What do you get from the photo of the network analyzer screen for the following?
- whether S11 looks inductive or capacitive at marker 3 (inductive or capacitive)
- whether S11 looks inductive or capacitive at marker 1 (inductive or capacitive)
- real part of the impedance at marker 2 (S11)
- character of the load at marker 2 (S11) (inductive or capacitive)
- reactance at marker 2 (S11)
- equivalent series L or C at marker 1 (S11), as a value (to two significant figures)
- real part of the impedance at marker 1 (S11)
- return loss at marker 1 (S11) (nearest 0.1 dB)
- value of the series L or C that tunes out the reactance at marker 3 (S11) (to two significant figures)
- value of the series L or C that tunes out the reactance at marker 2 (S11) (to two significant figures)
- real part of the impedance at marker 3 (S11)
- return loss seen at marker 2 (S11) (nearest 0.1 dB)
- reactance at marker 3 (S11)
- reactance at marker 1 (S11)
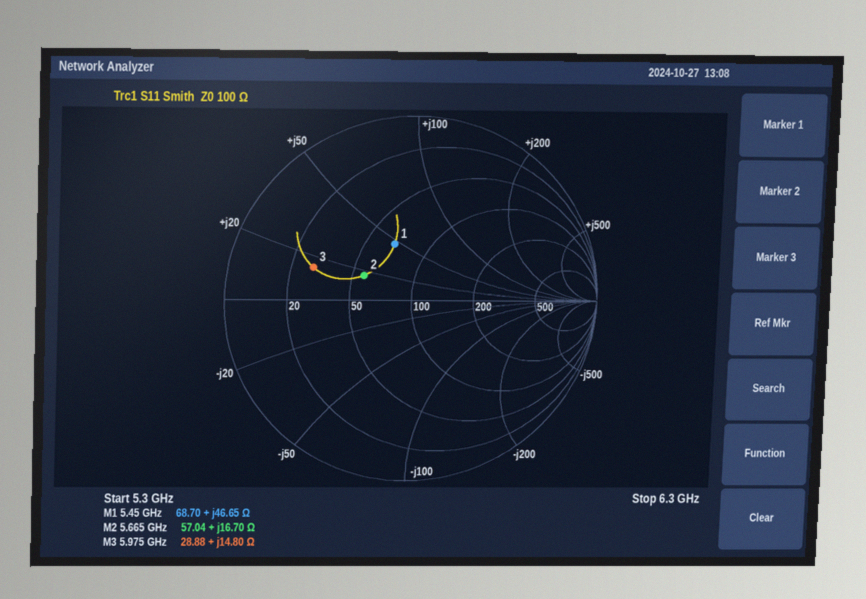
inductive
inductive
57.04 Ω
inductive
+16.70 Ω
1.4 nH
68.70 Ω
9.9 dB
1.8 pF
1.7 pF
28.88 Ω
10.7 dB
+14.80 Ω
+46.65 Ω
